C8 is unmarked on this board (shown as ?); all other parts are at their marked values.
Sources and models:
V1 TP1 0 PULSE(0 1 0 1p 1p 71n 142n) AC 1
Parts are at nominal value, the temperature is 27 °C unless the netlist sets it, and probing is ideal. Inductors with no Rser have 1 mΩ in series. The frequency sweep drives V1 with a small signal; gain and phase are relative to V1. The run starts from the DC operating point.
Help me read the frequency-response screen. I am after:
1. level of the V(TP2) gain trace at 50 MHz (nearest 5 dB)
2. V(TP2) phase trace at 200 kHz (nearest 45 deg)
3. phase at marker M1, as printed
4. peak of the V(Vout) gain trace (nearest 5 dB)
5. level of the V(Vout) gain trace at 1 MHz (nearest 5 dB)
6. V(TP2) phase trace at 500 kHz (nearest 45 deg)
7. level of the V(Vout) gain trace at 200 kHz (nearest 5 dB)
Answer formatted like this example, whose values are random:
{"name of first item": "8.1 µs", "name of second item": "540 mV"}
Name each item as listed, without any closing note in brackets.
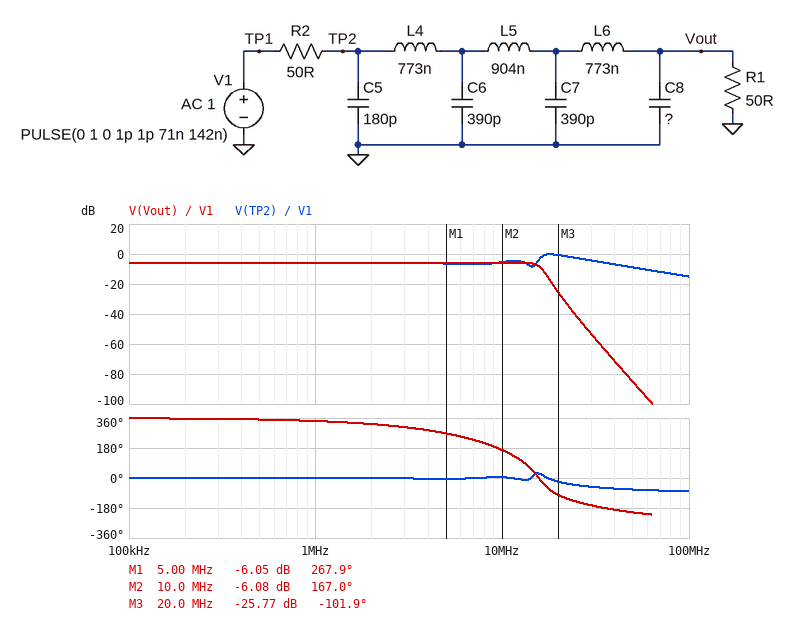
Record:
{"level of the V(TP2) gain trace at 50 MHz": "-10 dB", "V(TP2) phase trace at 200 kHz": "0 deg", "phase at marker M1, as printed": "267.9 deg", "peak of the V(Vout) gain trace": "-5 dB", "level of the V(Vout) gain trace at 1 MHz": "-5 dB", "V(TP2) phase trace at 500 kHz": "0 deg", "level of the V(Vout) gain trace at 200 kHz": "-5 dB"}
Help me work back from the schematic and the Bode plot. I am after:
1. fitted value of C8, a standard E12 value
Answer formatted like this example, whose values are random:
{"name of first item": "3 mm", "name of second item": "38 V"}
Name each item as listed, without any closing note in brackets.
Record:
{"fitted value of C8, a standard E12 value": "82 pF"}
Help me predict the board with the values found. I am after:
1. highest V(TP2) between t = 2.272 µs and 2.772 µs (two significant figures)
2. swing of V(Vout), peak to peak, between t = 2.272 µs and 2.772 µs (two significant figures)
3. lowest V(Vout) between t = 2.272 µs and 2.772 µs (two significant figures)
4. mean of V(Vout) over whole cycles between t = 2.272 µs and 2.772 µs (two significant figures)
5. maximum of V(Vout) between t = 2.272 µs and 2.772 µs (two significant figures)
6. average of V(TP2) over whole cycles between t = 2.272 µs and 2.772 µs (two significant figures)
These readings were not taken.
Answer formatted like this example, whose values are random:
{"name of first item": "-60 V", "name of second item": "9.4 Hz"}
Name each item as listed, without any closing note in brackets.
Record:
{"highest V(TP2) between t = 2.272 µs and 2.772 µs": "630 mV", "swing of V(Vout), peak to peak, between t = 2.272 µs and 2.772 µs": "630 mV", "lowest V(Vout) between t = 2.272 µs and 2.772 µs": "-66 mV", "mean of V(Vout) over whole cycles between t = 2.272 µs and 2.772 µs": "250 mV", "maximum of V(Vout) between t = 2.272 µs and 2.772 µs": "570 mV", "average of V(TP2) over whole cycles between t = 2.272 µs and 2.772 µs": "250 mV"}
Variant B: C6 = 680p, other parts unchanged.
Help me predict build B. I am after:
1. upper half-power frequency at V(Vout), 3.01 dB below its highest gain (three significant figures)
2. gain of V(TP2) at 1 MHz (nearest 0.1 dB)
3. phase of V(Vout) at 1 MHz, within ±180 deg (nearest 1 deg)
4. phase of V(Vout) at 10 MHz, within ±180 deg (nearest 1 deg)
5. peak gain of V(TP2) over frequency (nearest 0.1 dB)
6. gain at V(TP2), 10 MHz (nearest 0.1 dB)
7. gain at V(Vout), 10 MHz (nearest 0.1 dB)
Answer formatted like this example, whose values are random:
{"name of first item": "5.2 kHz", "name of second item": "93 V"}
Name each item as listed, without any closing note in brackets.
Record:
{"upper half-power frequency at V(Vout), 3.01 dB below its highest gain": "13.5 MHz", "gain of V(TP2) at 1 MHz": "-6.1 dB", "phase of V(Vout) at 1 MHz, within ±180 deg": "-21 deg", "phase of V(Vout) at 10 MHz, within ±180 deg": "142 deg", "peak gain of V(TP2) over frequency": "-0.1 dB", "gain at V(TP2), 10 MHz": "-5.9 dB", "gain at V(Vout), 10 MHz": "-6.9 dB"}
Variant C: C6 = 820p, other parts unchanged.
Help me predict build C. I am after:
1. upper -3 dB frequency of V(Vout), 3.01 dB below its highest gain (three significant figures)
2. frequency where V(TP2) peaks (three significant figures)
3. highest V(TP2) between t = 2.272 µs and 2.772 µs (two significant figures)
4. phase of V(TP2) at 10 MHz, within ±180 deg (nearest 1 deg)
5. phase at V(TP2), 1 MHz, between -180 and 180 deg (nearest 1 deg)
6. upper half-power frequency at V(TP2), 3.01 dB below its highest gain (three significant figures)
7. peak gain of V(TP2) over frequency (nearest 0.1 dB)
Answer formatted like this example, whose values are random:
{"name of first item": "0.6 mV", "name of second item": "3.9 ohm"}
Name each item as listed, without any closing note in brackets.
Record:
{"upper -3 dB frequency of V(Vout), 3.01 dB below its highest gain": "12.5 MHz", "frequency where V(TP2) peaks": "15.7 MHz", "highest V(TP2) between t = 2.272 µs and 2.772 µs": "610 mV", "phase of V(TP2) at 10 MHz, within ±180 deg": "31 deg", "phase at V(TP2), 1 MHz, between -180 and 180 deg": "-4 deg", "upper half-power frequency at V(TP2), 3.01 dB below its highest gain": "25.7 MHz", "peak gain of V(TP2) over frequency": "-0.1 dB"}
